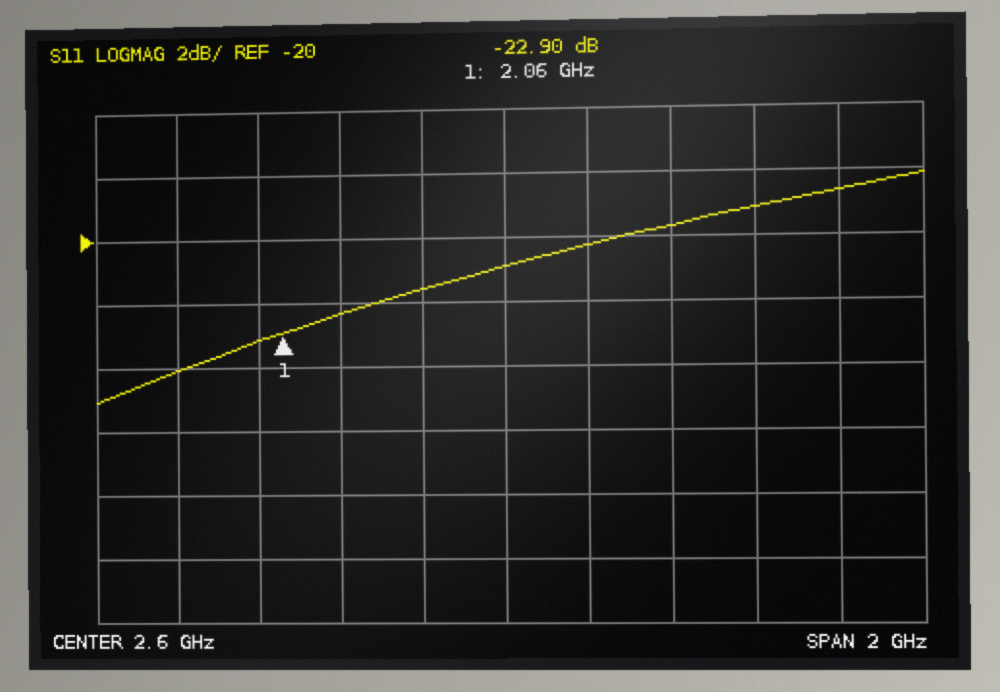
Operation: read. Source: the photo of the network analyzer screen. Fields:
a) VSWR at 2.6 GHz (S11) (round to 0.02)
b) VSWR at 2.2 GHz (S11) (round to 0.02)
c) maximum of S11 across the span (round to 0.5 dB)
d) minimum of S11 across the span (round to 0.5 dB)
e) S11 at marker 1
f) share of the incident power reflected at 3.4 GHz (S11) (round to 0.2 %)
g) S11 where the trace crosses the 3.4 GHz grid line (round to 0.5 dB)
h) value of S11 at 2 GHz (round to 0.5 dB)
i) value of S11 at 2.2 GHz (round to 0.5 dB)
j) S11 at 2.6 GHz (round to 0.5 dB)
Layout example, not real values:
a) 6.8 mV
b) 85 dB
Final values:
a) 1.20
b) 1.16
c) -18.0 dB
d) -25.0 dB
e) -22.90 dB
f) 1.4 %
g) -18.5 dB
h) -23.0 dB
i) -22.5 dB
j) -21.0 dB
